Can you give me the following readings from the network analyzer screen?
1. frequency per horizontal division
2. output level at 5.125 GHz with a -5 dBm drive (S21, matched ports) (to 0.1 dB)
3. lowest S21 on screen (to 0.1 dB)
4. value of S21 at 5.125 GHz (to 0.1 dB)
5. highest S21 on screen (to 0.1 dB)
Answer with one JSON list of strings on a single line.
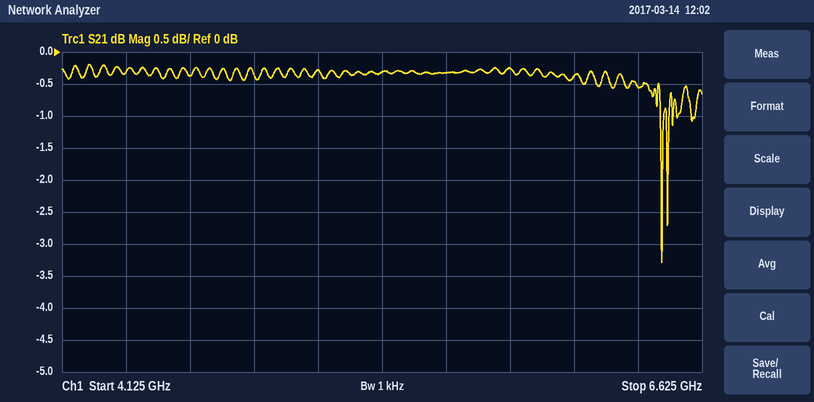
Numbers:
["250 MHz", "-5.3 dBm", "-3.3 dB", "-0.3 dB", "-0.2 dB"]
